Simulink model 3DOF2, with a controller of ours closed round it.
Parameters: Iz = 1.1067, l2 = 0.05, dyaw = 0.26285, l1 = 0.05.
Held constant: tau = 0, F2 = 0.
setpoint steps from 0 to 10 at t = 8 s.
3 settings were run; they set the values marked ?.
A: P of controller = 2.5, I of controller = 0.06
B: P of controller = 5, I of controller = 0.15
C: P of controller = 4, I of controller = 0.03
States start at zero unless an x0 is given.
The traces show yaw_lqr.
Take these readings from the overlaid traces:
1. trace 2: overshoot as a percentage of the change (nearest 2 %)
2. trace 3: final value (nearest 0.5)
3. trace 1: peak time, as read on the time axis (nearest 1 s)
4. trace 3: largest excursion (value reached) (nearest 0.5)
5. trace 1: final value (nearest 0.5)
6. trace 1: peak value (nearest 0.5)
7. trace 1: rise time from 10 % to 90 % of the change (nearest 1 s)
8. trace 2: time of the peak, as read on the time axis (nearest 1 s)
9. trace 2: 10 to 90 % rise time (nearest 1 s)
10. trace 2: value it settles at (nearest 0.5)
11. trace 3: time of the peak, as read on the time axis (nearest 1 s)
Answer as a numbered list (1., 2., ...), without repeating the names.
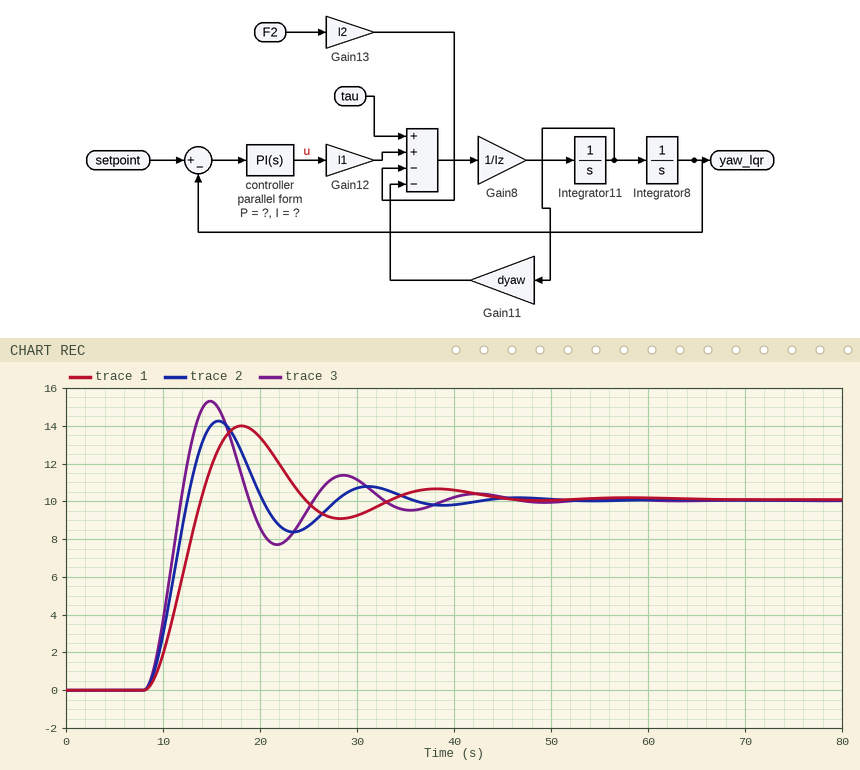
1. 42 %
2. 10.0
3. 18 s
4. 15.5
5. 10.0
6. 14.0
7. 4 s
8. 16 s
9. 3 s
10. 10.0
11. 15 s
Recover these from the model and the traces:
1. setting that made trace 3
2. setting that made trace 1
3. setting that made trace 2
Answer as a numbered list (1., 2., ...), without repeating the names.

1. B
2. A
3. C
